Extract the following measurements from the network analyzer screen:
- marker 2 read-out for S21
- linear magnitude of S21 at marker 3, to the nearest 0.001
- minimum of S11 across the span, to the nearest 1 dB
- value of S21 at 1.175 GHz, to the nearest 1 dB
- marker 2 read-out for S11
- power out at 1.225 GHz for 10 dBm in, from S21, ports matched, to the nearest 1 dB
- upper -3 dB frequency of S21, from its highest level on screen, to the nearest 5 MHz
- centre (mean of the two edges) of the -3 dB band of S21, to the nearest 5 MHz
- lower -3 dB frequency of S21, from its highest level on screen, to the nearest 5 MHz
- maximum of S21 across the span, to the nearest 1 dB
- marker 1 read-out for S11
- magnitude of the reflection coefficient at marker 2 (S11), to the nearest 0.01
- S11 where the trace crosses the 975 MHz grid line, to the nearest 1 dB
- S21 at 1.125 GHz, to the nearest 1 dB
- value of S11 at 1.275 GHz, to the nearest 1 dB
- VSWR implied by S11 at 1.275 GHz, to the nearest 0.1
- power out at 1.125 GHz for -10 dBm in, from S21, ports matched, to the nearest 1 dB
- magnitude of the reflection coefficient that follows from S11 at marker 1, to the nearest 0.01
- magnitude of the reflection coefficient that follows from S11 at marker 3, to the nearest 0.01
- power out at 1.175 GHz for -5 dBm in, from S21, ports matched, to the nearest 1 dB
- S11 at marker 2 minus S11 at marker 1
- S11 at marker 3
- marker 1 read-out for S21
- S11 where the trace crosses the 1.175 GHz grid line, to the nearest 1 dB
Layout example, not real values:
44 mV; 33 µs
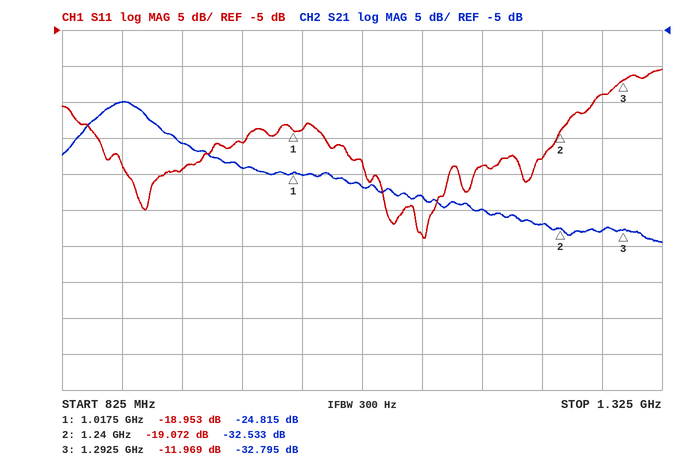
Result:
-32.533 dB; 0.023; -34 dB; -30 dB; -19.072 dB; -22 dBm; 900 MHz; 875 MHz; 850 MHz; -15 dB; -18.953 dB; 0.11; -21 dB; -28 dB; -14 dB; 1.5; -38 dBm; 0.11; 0.25; -35 dBm; -0.119 dB; -11.969 dB; -24.815 dB; -24 dB
